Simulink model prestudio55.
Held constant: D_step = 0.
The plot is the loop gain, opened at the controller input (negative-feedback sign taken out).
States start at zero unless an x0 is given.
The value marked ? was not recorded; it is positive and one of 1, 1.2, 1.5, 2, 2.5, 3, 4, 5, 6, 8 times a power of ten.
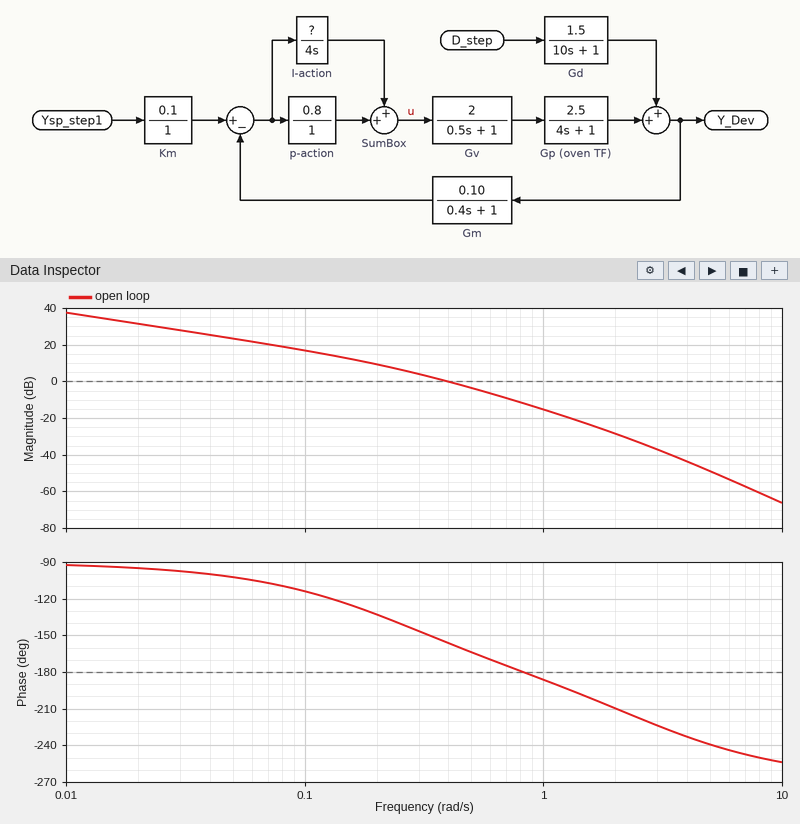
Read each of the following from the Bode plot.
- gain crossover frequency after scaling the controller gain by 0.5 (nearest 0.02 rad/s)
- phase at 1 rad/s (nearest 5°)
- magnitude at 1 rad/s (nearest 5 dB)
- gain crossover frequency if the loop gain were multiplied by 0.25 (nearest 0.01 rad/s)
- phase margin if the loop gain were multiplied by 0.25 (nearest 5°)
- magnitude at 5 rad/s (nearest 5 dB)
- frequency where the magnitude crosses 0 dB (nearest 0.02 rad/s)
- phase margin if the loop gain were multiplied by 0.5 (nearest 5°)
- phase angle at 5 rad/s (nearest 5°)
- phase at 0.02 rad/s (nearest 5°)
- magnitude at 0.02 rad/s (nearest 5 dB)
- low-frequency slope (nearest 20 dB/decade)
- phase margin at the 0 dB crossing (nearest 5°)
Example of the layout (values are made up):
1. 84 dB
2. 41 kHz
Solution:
1. 0.26 rad/s
2. -185°
3. -15 dB
4. 0.16 rad/s
5. 55°
6. -50 dB
7. 0.40 rad/s
8. 40°
9. -240°
10. -95°
11. 30 dB
12. -20 dB/decade
13. 25°
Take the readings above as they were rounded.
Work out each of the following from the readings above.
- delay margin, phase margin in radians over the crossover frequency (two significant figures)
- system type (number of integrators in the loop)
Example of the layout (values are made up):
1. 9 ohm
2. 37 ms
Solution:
1. 1.1 s
2. 1
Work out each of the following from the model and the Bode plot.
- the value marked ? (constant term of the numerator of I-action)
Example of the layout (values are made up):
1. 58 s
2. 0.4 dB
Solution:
1. 6
